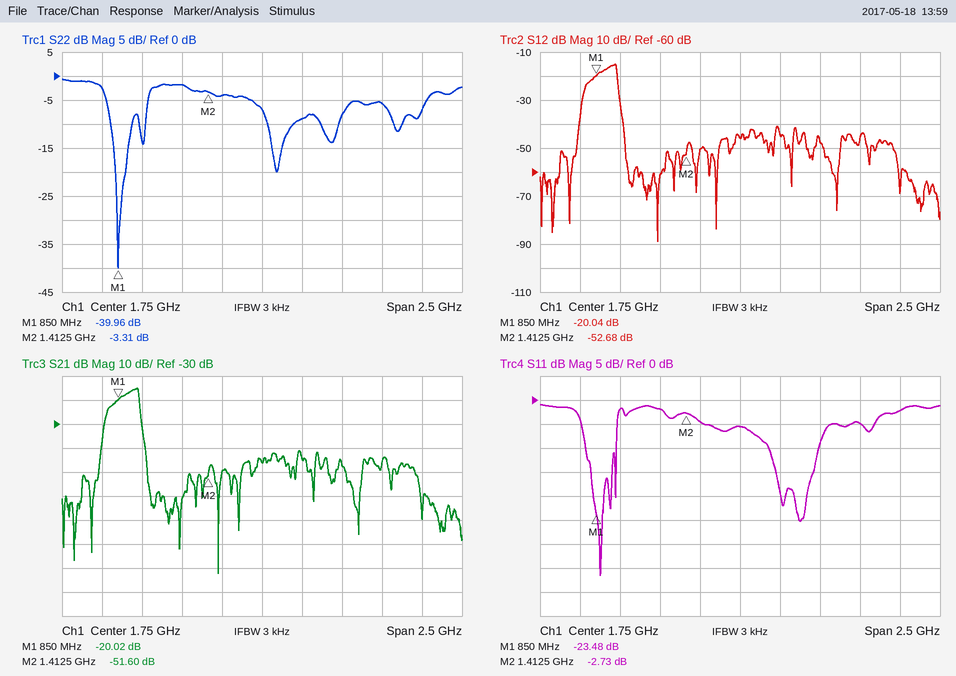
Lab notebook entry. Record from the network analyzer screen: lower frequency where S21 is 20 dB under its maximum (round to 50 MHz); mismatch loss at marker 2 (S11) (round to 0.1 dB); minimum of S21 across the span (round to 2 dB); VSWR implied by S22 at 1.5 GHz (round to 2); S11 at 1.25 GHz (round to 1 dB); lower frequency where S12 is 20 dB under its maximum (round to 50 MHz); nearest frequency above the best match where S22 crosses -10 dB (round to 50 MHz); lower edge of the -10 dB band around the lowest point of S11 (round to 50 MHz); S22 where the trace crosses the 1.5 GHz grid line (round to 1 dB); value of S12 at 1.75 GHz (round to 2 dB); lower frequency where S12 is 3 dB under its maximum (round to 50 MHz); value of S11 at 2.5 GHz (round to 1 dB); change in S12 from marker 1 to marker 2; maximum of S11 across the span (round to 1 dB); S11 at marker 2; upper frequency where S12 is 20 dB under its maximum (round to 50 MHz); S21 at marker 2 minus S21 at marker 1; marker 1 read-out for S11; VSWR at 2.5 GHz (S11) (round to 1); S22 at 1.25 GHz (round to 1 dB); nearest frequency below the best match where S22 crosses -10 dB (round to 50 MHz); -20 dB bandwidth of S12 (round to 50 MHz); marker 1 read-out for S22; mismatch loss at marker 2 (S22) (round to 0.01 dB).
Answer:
750 MHz
3.3 dB
-92 dB
4
-2 dB
750 MHz
950 MHz
800 MHz
-4 dB
-46 dB
900 MHz
-5 dB
-32.64 dB
-1 dB
-2.73 dB
1.00 GHz
-31.58 dB
-23.48 dB
4
-2 dB
800 MHz
250 MHz
-39.96 dB
2.73 dB
